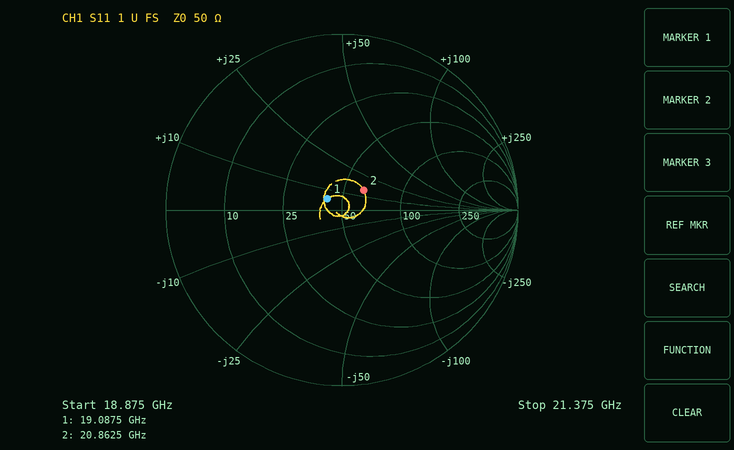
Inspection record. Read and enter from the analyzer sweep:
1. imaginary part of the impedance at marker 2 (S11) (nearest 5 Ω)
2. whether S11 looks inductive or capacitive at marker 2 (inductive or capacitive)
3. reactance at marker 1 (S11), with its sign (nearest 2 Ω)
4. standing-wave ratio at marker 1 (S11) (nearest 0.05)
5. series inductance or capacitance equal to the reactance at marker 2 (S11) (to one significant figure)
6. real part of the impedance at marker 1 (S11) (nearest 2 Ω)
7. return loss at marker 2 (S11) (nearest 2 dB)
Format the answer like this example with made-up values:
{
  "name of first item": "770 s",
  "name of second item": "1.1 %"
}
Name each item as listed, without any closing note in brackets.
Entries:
{
  "imaginary part of the impedance at marker 2 (S11)": "+15 Ω",
  "whether S11 looks inductive or capacitive at marker 2": "inductive",
  "reactance at marker 1 (S11), with its sign": "+6 Ω",
  "standing-wave ratio at marker 1 (S11)": "1.25",
  "series inductance or capacitance equal to the reactance at marker 2 (S11)": "100 pH",
  "real part of the impedance at marker 1 (S11)": "42 Ω",
  "return loss at marker 2 (S11)": "16 dB"
}
